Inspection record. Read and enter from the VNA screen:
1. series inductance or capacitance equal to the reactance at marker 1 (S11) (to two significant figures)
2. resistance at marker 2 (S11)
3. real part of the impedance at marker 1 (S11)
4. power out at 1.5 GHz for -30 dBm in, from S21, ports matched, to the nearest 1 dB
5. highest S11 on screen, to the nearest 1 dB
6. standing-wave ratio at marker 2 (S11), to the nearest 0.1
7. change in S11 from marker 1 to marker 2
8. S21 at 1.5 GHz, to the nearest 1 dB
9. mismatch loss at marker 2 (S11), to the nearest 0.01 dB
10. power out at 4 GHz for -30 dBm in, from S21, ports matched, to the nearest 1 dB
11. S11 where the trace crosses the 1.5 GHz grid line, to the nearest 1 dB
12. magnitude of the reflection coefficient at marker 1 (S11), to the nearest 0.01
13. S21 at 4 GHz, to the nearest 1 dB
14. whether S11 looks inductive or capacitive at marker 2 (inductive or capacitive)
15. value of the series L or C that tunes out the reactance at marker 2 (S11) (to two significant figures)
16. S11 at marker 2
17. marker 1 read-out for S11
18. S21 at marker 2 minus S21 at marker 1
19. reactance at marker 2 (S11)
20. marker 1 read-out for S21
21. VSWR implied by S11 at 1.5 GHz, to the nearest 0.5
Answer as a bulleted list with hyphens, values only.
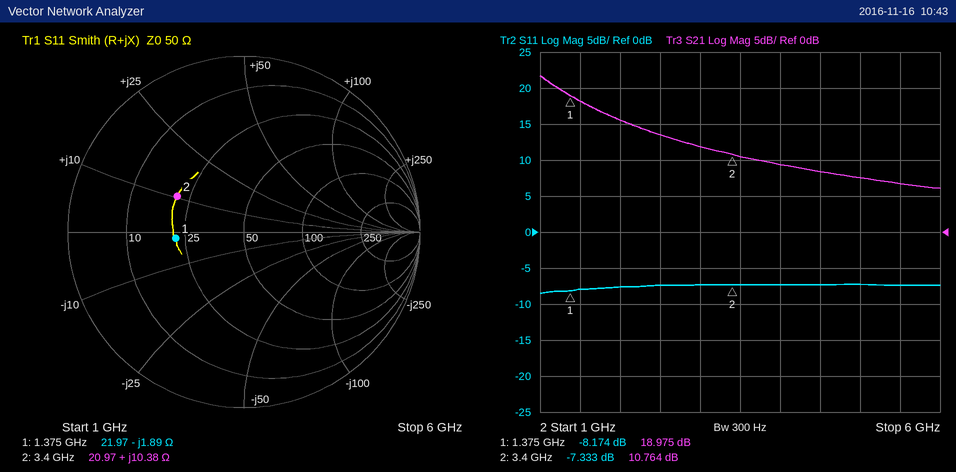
- 61 pF
- 20.97 Ω
- 21.97 Ω
- -12 dBm
- -7 dB
- 2.5
- 0.841 dB
- 18 dB
- 0.89 dB
- -21 dBm
- -8 dB
- 0.39
- 9 dB
- inductive
- 4.5 pF
- -7.333 dB
- -8.174 dB
- -8.211 dB
- +10.38 Ω
- 18.975 dB
- 2.5
